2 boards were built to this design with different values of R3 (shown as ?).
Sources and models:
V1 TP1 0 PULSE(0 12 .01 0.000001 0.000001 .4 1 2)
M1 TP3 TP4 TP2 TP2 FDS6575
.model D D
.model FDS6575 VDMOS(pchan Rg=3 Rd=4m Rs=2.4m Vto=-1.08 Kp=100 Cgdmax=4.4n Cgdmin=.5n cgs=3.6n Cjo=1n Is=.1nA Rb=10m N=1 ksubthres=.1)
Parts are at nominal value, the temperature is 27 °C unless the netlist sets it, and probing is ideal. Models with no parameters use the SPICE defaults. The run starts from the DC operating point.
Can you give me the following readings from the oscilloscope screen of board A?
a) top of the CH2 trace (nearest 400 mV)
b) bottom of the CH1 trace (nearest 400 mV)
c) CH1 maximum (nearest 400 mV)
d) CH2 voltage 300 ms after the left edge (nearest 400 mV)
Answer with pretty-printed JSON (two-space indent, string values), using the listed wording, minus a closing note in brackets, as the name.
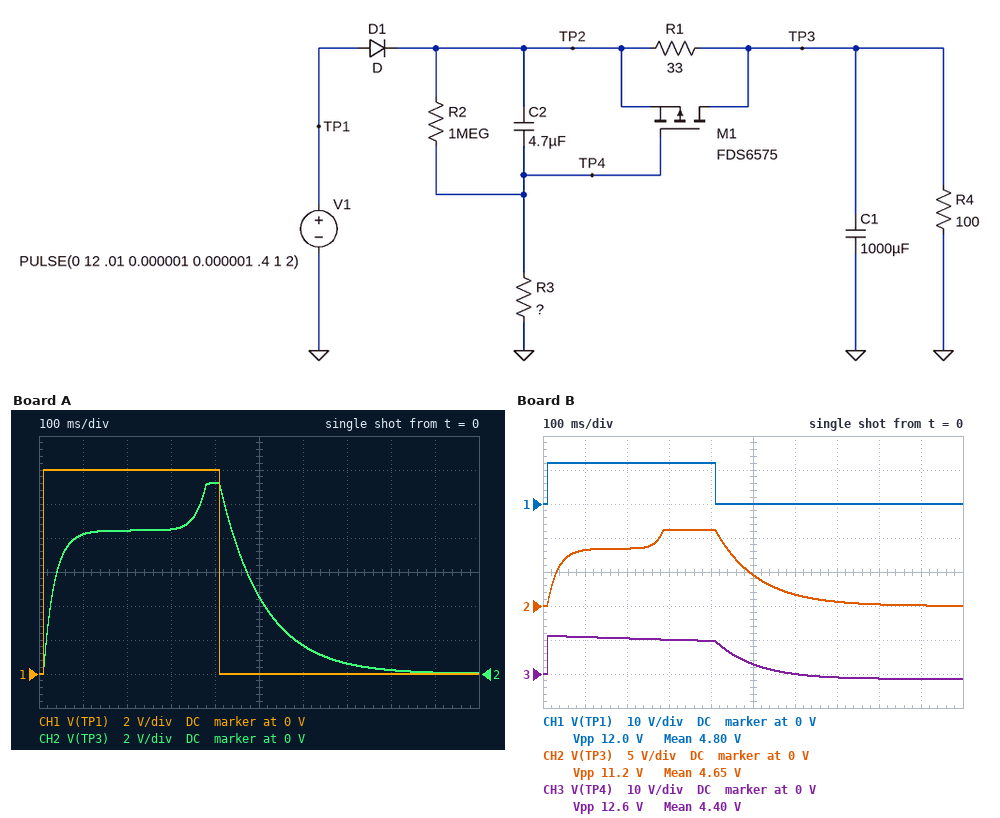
{
  "top of the CH2 trace": "11.2 V",
  "bottom of the CH1 trace": "0 V",
  "CH1 maximum": "12.0 V",
  "CH2 voltage 300 ms after the left edge": "8.4 V"
}
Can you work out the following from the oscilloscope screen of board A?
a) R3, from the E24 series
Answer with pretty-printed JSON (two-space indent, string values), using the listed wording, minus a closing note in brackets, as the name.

{
  "R3, from the E24 series": "750 kΩ"
}
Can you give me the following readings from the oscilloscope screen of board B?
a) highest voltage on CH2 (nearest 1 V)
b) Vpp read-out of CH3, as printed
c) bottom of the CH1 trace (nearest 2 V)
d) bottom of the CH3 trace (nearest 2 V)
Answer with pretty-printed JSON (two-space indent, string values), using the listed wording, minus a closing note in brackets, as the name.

{
  "highest voltage on CH2": "11 V",
  "Vpp read-out of CH3, as printed": "12.6 V",
  "bottom of the CH1 trace": "0 V",
  "bottom of the CH3 trace": "-2 V"
}
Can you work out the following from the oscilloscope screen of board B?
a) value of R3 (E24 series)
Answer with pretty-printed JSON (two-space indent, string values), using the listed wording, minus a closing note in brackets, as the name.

{
  "value of R3": "560 kΩ"
}
